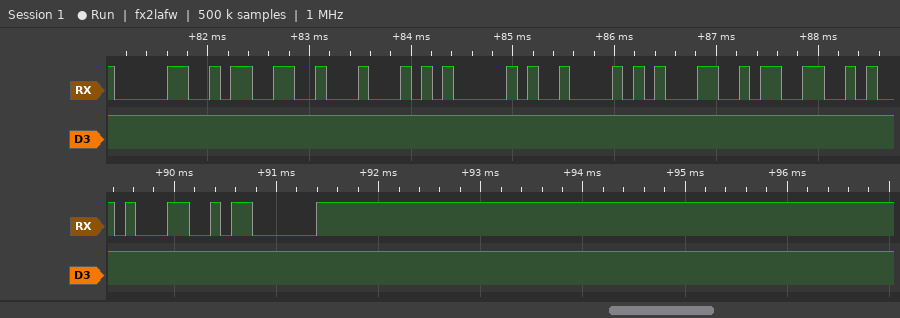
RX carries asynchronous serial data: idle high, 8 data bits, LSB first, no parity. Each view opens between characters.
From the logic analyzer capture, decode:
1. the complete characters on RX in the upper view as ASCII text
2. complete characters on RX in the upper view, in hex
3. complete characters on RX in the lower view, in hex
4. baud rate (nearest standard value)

"03DAB13"
30, 33, 44, 41, 42, 31, 33
31, 03
9600 baud
